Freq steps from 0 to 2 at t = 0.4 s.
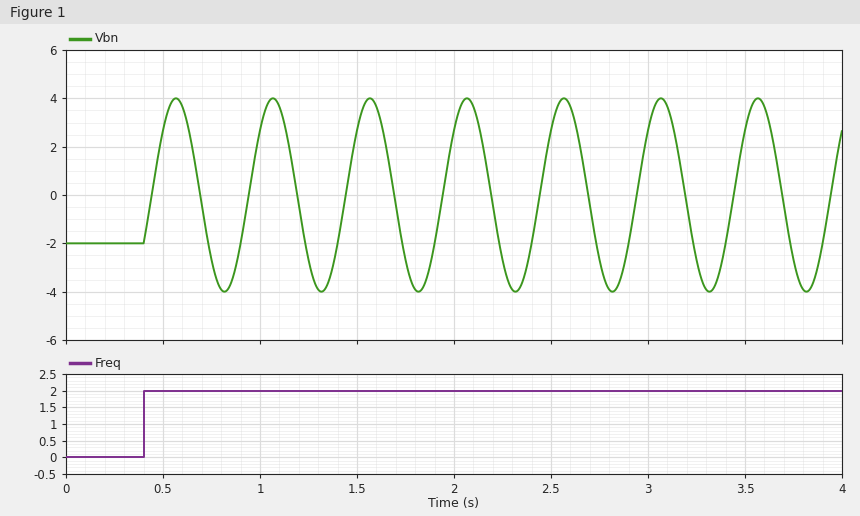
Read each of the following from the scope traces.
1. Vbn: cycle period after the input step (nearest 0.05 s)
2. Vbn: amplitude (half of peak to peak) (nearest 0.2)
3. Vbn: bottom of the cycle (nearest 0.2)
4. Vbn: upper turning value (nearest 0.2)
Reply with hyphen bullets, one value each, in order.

- 0.50 s
- 4.0
- -4.0
- 4.0
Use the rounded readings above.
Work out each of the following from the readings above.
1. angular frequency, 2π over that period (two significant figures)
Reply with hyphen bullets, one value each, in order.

- 13 rad/s
